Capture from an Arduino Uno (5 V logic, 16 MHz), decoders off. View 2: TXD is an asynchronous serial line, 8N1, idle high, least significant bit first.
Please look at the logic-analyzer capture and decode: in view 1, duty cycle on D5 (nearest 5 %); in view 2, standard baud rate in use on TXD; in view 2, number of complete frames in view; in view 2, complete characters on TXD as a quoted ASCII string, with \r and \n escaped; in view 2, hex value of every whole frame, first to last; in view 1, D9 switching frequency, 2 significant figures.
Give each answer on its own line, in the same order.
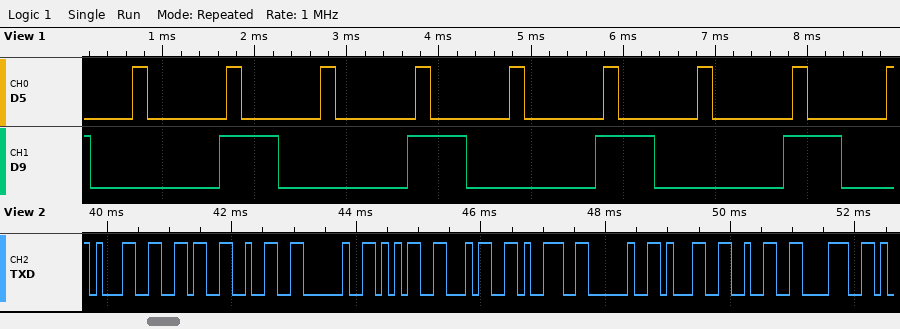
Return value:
15 %
9600 baud
11
"162 549 128"
31 36 32 20 35 34 39 20 31 32 38
490 Hz
